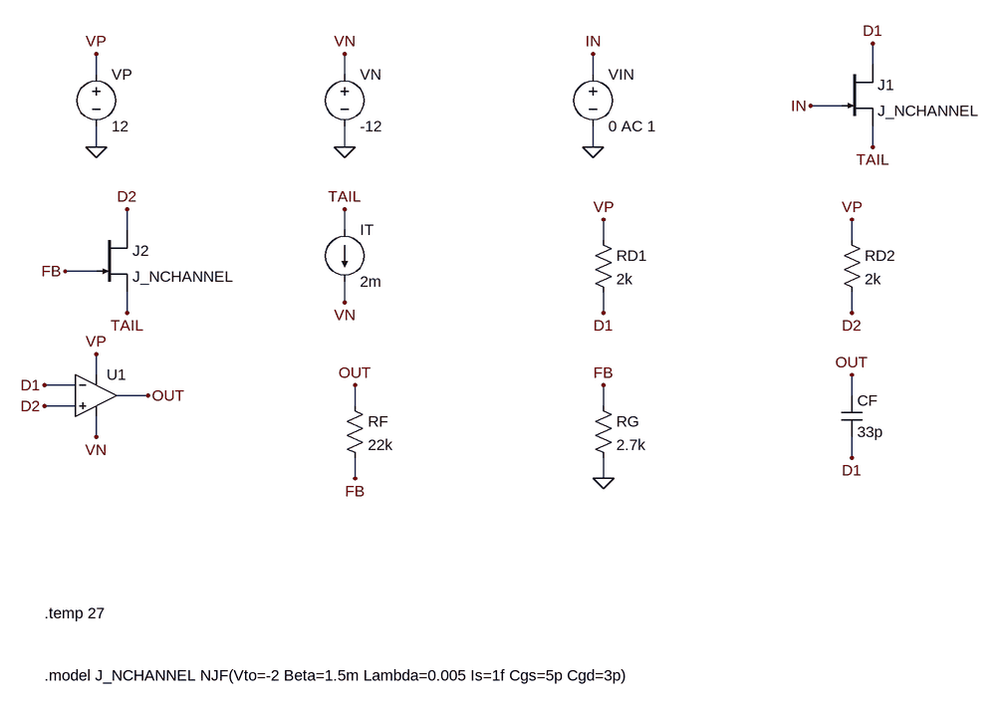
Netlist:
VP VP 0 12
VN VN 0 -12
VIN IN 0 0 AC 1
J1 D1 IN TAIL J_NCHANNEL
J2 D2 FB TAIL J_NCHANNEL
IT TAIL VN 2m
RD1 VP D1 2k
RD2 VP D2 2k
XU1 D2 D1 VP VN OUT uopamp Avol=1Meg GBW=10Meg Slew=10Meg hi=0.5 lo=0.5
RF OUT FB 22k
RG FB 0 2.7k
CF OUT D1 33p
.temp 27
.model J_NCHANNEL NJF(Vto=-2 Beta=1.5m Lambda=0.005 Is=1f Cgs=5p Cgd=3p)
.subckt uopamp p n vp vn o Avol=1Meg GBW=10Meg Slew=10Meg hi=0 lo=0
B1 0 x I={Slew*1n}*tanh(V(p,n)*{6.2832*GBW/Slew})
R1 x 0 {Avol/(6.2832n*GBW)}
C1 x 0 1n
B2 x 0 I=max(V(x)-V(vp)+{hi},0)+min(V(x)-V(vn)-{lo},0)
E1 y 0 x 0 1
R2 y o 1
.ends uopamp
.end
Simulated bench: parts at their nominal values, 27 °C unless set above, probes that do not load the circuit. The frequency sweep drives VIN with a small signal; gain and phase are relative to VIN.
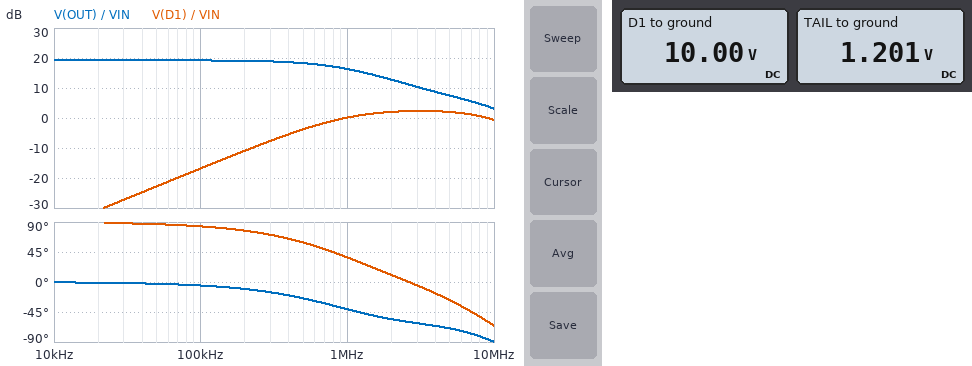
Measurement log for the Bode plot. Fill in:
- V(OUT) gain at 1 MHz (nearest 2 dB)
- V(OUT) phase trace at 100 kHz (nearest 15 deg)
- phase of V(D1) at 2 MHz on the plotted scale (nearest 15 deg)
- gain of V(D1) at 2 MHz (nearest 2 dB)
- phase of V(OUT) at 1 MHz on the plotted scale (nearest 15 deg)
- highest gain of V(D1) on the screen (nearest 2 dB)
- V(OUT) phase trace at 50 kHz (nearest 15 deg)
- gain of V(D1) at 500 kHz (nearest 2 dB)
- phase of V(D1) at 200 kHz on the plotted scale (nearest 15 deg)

16 dB
0 deg
15 deg
2 dB
-45 deg
2 dB
0 deg
-4 dB
75 deg
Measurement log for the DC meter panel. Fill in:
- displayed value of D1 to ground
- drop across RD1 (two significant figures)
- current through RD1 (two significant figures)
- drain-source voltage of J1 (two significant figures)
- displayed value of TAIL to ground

10.00 V
2.0 V
1.0 mA
8.8 V
1.201 V
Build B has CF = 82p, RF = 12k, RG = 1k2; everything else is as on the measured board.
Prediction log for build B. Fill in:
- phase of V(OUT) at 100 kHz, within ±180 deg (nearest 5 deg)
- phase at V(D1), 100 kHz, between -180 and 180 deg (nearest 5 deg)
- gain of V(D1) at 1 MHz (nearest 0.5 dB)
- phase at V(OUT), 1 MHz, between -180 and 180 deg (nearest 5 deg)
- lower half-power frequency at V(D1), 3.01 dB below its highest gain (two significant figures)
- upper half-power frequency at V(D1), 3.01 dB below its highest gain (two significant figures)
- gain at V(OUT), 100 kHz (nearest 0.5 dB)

-15 deg
75 deg
4.5 dB
-50 deg
330 kHz
12 MHz
20.5 dB
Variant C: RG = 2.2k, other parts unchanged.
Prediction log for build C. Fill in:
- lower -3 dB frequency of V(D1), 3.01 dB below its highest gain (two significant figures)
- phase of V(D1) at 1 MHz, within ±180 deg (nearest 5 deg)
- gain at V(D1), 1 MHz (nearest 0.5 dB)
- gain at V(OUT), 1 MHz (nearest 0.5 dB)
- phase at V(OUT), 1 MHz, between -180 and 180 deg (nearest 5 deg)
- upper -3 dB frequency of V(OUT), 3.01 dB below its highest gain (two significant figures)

720 kHz
30 deg
1.0 dB
17.0 dB
-45 deg
850 kHz
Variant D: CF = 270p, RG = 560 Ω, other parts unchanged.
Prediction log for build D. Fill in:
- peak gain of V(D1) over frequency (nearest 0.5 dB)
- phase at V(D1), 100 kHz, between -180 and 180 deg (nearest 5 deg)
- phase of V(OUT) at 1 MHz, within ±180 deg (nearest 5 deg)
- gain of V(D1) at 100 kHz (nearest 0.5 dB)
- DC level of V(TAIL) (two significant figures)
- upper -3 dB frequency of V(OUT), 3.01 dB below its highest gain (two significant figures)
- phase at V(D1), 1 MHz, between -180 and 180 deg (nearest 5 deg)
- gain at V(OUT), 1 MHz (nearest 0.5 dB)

7.0 dB
20 deg
-35 deg
6.5 dB
1.2 V
34 kHz
-5 deg
8.5 dB
